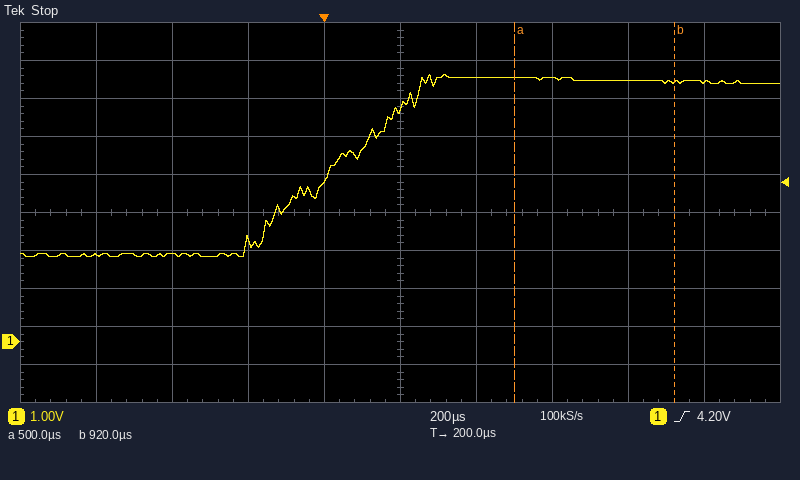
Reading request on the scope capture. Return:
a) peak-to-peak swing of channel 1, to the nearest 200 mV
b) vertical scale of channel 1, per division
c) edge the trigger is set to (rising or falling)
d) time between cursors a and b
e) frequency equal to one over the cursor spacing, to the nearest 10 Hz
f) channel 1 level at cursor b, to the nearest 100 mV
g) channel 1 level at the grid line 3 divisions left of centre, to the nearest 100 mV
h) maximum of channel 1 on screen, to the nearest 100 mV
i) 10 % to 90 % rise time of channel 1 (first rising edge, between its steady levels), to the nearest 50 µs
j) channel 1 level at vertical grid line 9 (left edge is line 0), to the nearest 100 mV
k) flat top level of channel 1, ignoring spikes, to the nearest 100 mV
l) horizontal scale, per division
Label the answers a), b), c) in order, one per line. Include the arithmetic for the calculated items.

a) 4.8 V
b) 1 V
c) rising
d) 920 µs − (500 µs) = 420 µs
e) 1 / 420 µs ≈ 2.38 kHz
f) 6.8 V
g) 2.3 V
h) 7.0 V
i) 400 µs
j) 6.8 V
k) 6.9 V
l) 200 µs
